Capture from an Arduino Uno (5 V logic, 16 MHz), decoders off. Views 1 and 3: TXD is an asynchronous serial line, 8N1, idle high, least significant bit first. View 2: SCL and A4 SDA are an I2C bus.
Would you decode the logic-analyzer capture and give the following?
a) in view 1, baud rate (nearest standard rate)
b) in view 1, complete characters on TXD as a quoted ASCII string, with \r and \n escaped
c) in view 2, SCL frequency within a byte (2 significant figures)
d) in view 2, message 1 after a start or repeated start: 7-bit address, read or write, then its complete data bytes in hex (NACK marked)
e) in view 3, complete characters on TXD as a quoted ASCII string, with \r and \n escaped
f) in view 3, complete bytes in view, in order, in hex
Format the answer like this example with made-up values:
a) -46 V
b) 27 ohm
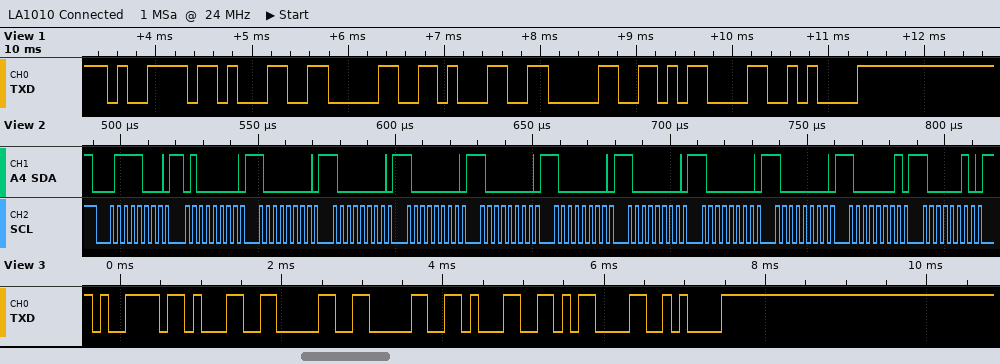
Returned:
a) 9600 baud
b) "y1010\r\n"
c) 400 kHz
d) 0x3C write: 40 80 80 80 80 80 80 80 80 81 82
e) "y1001\r\n"
f) 79 31 30 30 31 0D 0A
